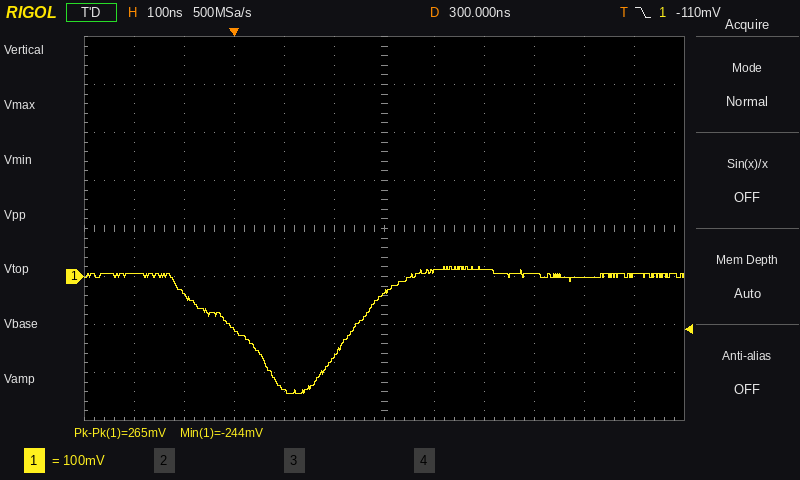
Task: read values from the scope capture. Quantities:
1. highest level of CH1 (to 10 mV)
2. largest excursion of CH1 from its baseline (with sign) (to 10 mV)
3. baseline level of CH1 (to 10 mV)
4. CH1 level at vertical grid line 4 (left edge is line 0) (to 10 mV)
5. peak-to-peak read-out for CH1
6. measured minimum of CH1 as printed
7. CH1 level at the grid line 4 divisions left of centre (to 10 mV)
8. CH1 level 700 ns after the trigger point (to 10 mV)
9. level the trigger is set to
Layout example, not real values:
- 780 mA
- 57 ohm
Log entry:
- 20 mV
- -250 mV
- 0 mV
- -240 mV
- 265 mV
- -244 mV
- -40 mV
- 0 mV
- -110 mV
